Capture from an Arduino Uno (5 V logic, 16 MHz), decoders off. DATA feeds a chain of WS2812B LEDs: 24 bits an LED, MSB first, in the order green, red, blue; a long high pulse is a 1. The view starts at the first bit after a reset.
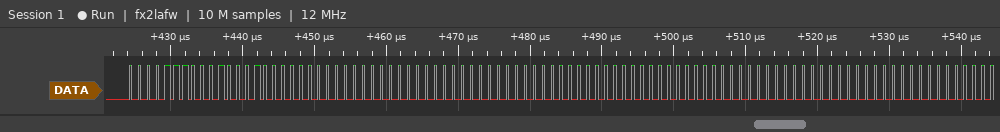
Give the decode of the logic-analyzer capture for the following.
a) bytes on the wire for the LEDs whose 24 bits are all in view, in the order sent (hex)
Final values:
0E 22 00 00 00 00 00 00 00 00 00 00
